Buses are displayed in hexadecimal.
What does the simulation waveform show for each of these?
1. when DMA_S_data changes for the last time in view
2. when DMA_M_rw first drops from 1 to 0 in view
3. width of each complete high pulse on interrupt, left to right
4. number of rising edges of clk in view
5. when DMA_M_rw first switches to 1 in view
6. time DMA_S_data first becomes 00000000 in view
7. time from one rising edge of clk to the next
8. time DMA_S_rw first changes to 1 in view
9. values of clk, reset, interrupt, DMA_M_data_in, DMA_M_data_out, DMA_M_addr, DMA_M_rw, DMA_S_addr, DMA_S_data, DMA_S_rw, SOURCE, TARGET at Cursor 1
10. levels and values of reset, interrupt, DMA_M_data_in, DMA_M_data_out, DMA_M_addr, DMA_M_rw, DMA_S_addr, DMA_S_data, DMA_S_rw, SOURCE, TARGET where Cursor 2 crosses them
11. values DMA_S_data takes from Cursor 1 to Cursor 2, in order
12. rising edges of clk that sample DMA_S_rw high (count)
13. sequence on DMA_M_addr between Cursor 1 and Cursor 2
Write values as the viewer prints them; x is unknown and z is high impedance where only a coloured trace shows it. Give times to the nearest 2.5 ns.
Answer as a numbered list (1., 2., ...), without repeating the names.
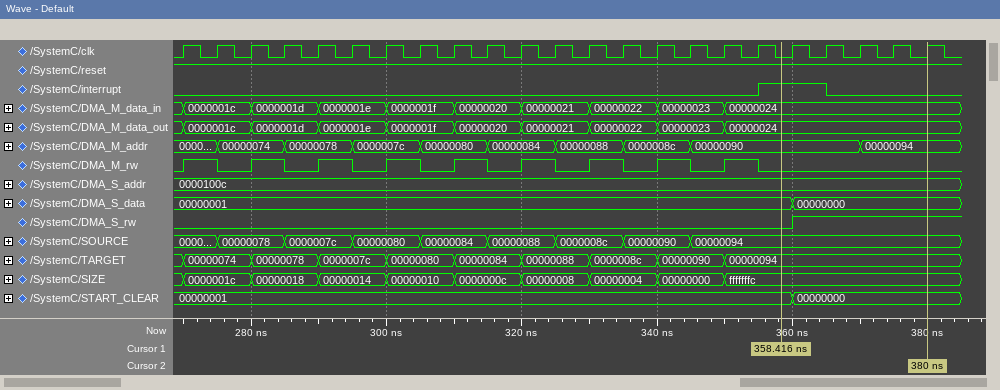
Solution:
1. 360 ns
2. 275 ns
3. 10 ns
4. 23
5. 270 ns
6. 360 ns
7. 5 ns
8. 360 ns
9. clk=0, reset=1, interrupt=1, DMA_M_data_in=00000024, DMA_M_data_out=00000024, DMA_M_addr=00000090, DMA_M_rw=0, DMA_S_addr=0000100c, DMA_S_data=00000001, DMA_S_rw=0, SOURCE=00000094, TARGET=00000094
10. reset=1, interrupt=0, DMA_M_data_in=00000024, DMA_M_data_out=00000024, DMA_M_addr=00000094, DMA_M_rw=0, DMA_S_addr=0000100c, DMA_S_data=00000000, DMA_S_rw=1, SOURCE=00000094, TARGET=00000094
11. 00000001, 00000000
12. 4
13. 00000090, 00000094
